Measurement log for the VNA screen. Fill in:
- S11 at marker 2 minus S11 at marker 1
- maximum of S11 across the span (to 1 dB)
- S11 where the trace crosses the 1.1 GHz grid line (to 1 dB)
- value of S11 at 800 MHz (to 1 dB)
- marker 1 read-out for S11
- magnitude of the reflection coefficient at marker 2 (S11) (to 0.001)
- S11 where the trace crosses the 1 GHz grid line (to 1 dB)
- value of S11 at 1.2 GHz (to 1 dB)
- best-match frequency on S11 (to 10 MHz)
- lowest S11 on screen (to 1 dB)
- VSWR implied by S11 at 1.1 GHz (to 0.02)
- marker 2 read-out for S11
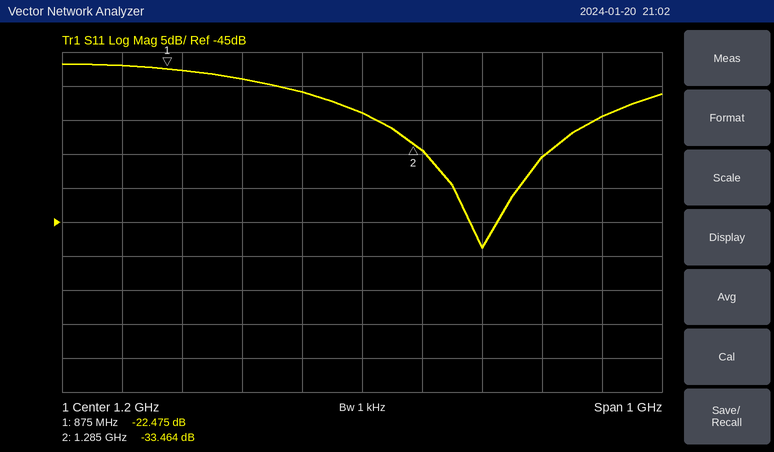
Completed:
-10.989 dB
-22 dB
-26 dB
-22 dB
-22.475 dB
0.021
-24 dB
-29 dB
1.40 GHz
-49 dB
1.10
-33.464 dB
